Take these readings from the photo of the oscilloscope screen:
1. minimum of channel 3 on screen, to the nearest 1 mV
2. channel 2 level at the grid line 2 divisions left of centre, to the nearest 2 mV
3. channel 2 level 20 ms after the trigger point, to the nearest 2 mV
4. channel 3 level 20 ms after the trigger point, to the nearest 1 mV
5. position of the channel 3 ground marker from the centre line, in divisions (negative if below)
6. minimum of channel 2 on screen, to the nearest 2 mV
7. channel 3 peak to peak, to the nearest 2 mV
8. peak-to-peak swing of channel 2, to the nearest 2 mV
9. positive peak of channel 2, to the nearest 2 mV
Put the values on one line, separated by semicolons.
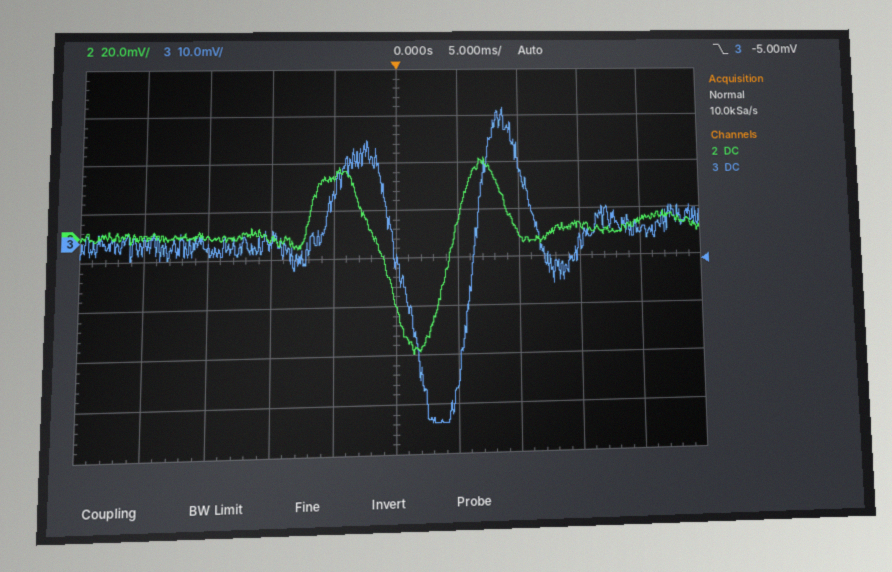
-38 mV; -2 mV; 4 mV; 1 mV; +0.4 div; -50 mV; 66 mV; 82 mV; 32 mV
